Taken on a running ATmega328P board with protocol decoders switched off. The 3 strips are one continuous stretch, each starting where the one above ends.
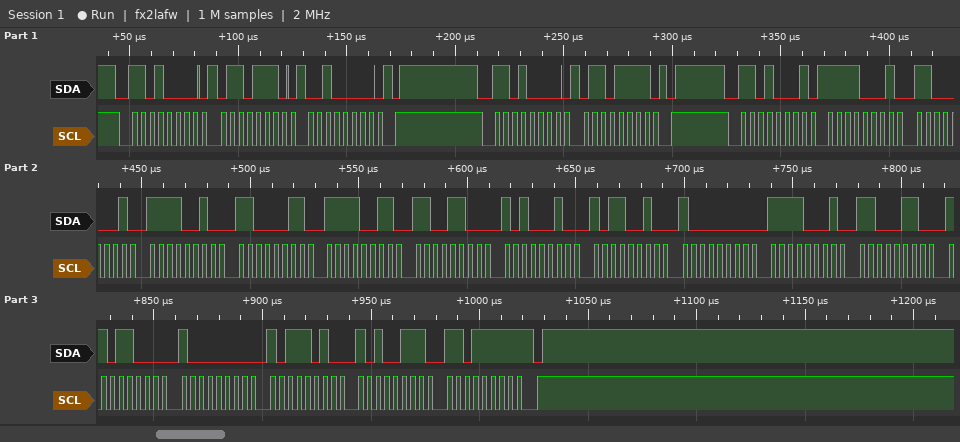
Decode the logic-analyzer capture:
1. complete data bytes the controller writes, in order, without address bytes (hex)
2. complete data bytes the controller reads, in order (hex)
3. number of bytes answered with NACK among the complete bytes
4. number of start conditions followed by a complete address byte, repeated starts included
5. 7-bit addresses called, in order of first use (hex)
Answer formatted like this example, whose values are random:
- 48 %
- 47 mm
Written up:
- 6E 20 6F
- F1 C1 F2 C3 F3 CC A2 B2 80 F1 C6 D8 80 BA A7 DF
- 1
- 3
- 0x68
